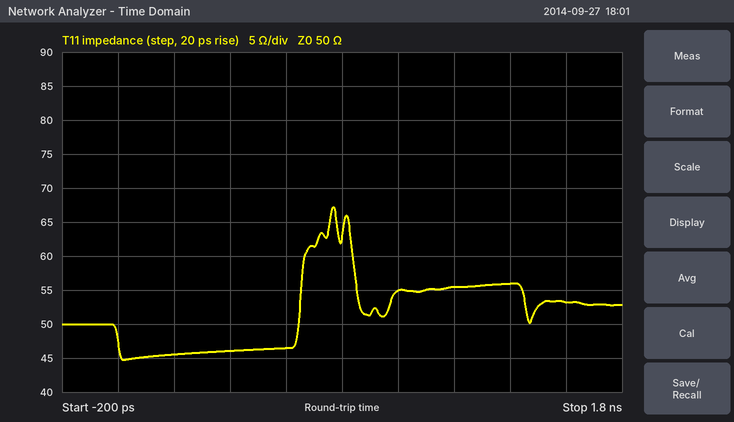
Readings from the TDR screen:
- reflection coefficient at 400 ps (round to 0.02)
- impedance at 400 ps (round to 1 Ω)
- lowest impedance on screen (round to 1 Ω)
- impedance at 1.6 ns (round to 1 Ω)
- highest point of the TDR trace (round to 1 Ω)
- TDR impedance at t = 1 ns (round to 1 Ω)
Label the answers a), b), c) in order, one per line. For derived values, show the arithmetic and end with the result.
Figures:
a) (46 − 50)/(46 + 50) ≈ -0.04
b) 46 Ω
c) 45 Ω
d) 53 Ω
e) 67 Ω
f) 55 Ω
